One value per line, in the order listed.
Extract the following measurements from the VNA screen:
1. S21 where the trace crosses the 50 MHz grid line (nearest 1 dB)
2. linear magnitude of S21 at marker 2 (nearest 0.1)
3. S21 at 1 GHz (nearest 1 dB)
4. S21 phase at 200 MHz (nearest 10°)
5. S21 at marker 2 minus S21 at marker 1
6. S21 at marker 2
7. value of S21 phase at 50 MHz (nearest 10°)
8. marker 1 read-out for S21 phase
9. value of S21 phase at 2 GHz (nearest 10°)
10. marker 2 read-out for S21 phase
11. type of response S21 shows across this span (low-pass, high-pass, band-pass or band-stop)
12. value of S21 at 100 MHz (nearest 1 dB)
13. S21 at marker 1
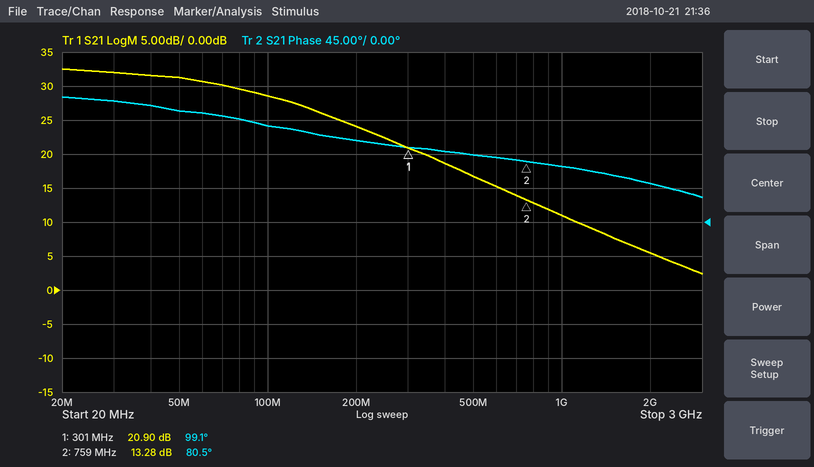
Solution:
31 dB
4.6
11 dB
110°
-7.62 dB
13.28 dB
150°
99.1°
50°
80.5°
low-pass
29 dB
20.90 dB
